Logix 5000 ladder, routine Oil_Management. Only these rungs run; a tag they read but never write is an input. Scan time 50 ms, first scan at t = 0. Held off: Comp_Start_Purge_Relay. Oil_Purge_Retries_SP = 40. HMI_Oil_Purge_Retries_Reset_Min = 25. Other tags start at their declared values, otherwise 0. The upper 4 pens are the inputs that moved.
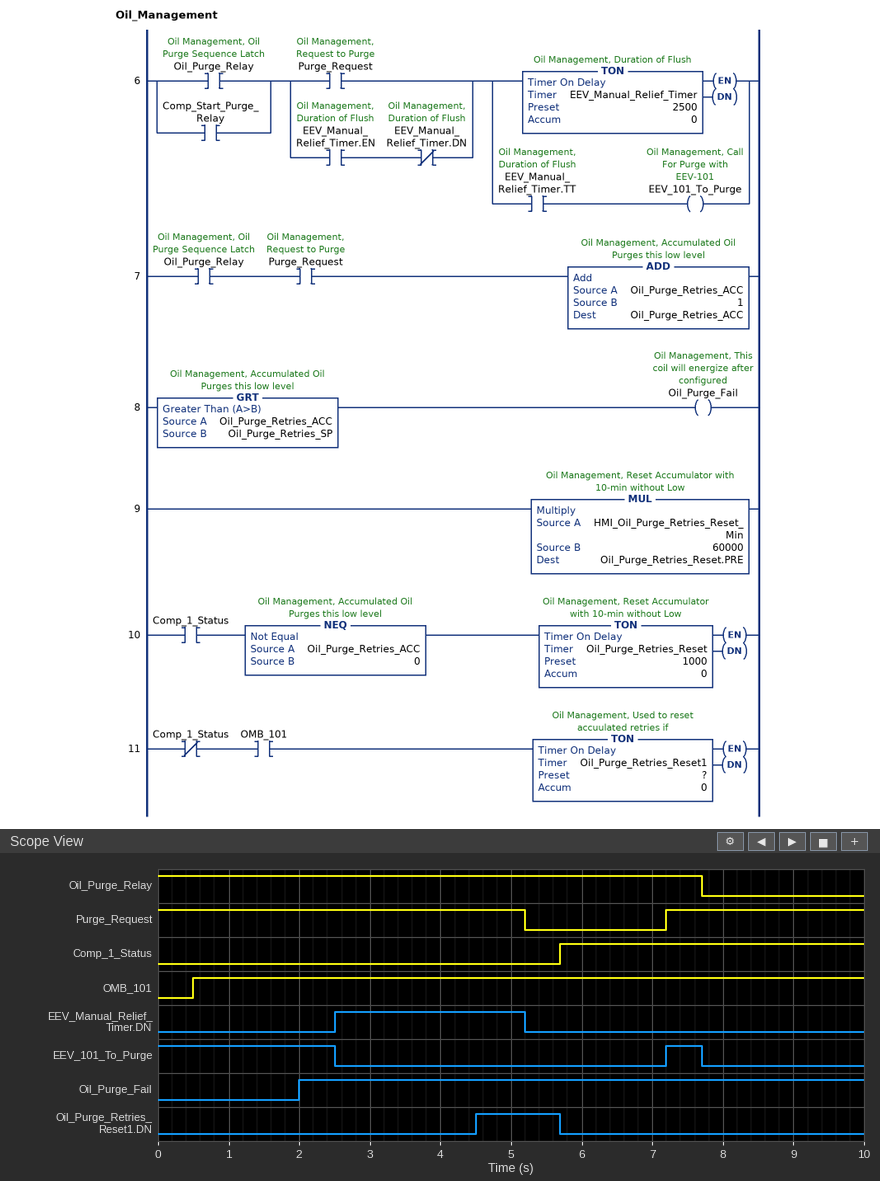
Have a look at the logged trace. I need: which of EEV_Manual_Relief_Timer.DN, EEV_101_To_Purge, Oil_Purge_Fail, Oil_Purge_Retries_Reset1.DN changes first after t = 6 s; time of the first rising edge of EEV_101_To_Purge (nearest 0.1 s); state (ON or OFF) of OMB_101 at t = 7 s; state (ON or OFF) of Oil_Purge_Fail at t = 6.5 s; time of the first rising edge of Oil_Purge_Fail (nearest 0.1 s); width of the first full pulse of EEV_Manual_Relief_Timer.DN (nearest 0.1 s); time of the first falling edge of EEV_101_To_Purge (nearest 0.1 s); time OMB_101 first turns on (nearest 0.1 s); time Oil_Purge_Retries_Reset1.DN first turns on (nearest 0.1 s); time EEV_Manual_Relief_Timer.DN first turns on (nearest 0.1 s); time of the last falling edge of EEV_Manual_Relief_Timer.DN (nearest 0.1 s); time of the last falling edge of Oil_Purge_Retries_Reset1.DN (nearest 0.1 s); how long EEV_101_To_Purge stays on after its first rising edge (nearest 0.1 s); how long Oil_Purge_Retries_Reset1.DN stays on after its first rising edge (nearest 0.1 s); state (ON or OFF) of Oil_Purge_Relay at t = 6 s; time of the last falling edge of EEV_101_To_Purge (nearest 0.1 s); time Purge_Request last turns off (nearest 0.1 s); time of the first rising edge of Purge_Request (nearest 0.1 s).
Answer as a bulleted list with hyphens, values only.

- EEV_101_To_Purge
- 7.2 s
- ON
- ON
- 2.0 s
- 2.7 s
- 2.5 s
- 0.5 s
- 4.5 s
- 2.5 s
- 5.2 s
- 5.7 s
- 0.5 s
- 1.2 s
- ON
- 7.7 s
- 5.2 s
- 7.2 s
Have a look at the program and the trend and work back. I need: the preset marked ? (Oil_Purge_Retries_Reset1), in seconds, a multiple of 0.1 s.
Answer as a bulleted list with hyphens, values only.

- 4.0 s
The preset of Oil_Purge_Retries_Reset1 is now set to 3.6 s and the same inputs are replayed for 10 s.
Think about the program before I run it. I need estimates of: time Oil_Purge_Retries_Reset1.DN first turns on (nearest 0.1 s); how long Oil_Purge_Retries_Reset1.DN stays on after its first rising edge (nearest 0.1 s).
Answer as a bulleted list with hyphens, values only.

- 4.1 s
- 1.6 s
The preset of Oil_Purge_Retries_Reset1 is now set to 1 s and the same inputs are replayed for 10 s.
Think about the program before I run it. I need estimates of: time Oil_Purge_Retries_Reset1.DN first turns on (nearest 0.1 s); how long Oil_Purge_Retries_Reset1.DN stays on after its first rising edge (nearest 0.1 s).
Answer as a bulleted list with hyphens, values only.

- 1.5 s
- 4.2 s
